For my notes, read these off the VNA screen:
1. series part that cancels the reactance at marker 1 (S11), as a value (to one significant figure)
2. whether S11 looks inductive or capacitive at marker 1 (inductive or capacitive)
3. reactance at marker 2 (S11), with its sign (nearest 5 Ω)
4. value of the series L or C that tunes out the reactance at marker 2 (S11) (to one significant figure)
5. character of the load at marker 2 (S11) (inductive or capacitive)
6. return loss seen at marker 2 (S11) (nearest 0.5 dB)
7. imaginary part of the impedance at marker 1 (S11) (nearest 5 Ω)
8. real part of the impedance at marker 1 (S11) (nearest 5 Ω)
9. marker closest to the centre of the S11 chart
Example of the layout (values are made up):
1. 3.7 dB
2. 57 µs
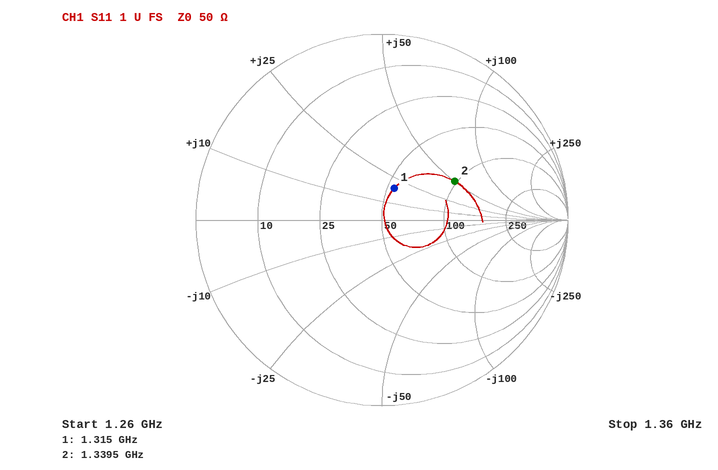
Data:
1. 6 pF
2. inductive
3. +50 Ω
4. 2 pF
5. inductive
6. 7.0 dB
7. +20 Ω
8. 55 Ω
9. marker 1
